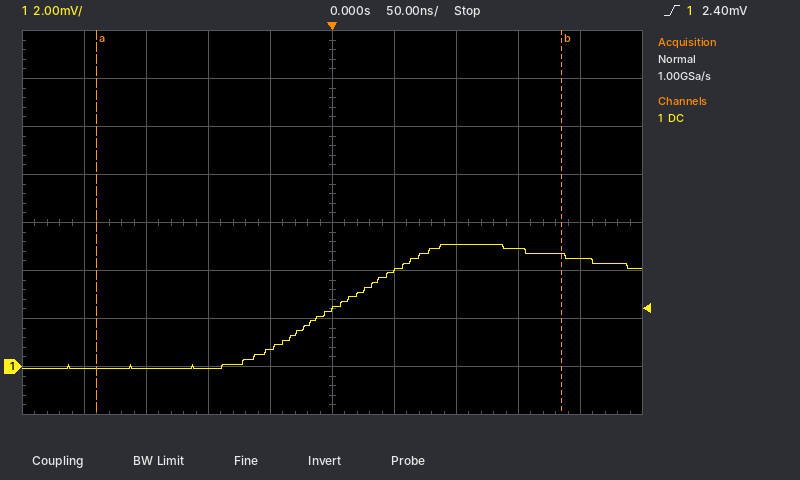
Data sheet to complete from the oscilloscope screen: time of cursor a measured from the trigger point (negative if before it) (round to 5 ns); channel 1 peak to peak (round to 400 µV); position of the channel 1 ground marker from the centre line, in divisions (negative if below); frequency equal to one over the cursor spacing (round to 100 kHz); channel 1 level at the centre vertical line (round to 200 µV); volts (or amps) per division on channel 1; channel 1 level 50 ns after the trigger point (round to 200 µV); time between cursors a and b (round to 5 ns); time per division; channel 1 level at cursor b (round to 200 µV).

-190 ns
5.2 mV
-3.0 div
2.7 MHz
2.4 mV
2 mV
4.0 mV
375 ns
50 ns
4.6 mV
